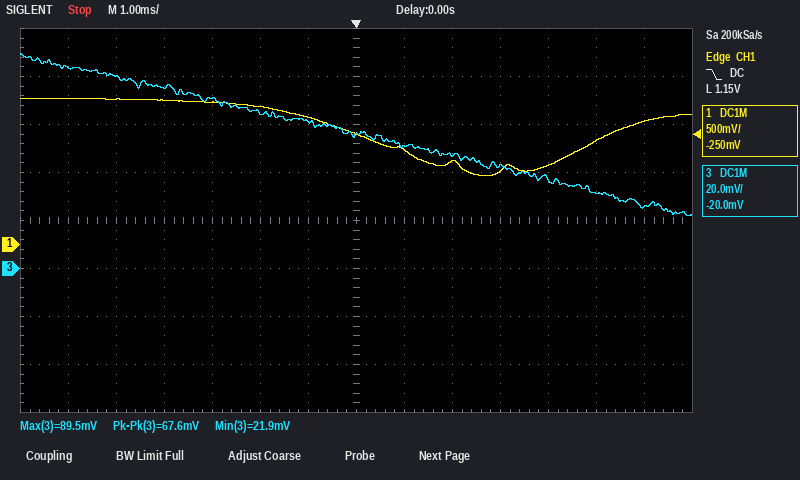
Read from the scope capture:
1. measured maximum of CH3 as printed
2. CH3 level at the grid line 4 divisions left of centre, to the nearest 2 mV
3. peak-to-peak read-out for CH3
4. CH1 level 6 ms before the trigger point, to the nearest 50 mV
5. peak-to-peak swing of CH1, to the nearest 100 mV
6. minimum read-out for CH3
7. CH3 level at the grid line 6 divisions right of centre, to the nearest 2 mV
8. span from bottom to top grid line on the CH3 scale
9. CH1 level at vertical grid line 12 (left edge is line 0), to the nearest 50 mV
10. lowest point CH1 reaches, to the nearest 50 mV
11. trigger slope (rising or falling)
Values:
89.5 mV
76 mV
67.6 mV
1.50 V
800 mV
21.9 mV
26 mV
160 mV
1.10 V
700 mV
falling
